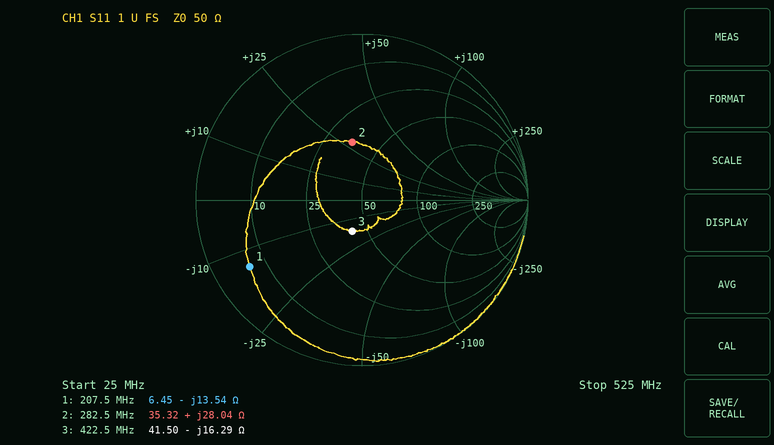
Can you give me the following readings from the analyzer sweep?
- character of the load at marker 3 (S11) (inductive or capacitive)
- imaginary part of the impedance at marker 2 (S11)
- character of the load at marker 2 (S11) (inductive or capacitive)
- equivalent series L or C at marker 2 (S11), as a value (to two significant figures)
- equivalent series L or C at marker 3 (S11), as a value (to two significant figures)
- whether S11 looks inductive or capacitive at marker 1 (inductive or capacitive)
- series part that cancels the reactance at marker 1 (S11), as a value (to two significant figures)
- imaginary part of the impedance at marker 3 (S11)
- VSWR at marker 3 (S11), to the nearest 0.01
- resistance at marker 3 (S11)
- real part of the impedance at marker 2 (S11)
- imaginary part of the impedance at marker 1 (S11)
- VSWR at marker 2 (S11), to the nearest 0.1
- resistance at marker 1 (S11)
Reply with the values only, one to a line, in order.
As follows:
capacitive
+28.04 Ω
inductive
16 nH
23 pF
capacitive
10 nH
-16.29 Ω
1.49
41.50 Ω
35.32 Ω
-13.54 Ω
2.1
6.45 Ω
